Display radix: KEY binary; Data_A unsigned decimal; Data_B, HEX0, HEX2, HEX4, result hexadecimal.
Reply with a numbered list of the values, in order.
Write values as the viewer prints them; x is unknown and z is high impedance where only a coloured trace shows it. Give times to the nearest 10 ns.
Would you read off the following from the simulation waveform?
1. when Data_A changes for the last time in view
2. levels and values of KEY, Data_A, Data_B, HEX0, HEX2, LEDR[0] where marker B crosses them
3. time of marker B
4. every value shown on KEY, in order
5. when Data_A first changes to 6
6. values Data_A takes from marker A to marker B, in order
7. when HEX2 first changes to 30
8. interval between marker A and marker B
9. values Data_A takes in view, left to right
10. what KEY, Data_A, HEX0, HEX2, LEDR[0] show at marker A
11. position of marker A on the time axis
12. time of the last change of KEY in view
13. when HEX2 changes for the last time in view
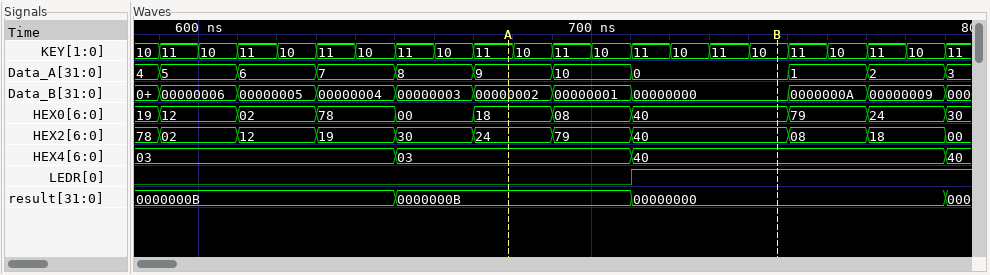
1. 790 ns
2. KEY=10, Data_A=0, Data_B=00000000, HEX0=40, HEX2=40, LEDR[0]=1
3. 750 ns
4. 10, 11, 10, 11, 10, 11, 10, 11, 10, 11, 10, 11, 10, 11, 10, 11, 10, 11, 10, 11, 10, 11
5. 610 ns
6. 9, 10, 0
7. 650 ns
8. 70 ns
9. 4, 5, 6, 7, 8, 9, 10, 0, 1, 2, 3
10. KEY=11, Data_A=9, HEX0=18, HEX2=24, LEDR[0]=0
11. 680 ns
12. 790 ns
13. 790 ns
